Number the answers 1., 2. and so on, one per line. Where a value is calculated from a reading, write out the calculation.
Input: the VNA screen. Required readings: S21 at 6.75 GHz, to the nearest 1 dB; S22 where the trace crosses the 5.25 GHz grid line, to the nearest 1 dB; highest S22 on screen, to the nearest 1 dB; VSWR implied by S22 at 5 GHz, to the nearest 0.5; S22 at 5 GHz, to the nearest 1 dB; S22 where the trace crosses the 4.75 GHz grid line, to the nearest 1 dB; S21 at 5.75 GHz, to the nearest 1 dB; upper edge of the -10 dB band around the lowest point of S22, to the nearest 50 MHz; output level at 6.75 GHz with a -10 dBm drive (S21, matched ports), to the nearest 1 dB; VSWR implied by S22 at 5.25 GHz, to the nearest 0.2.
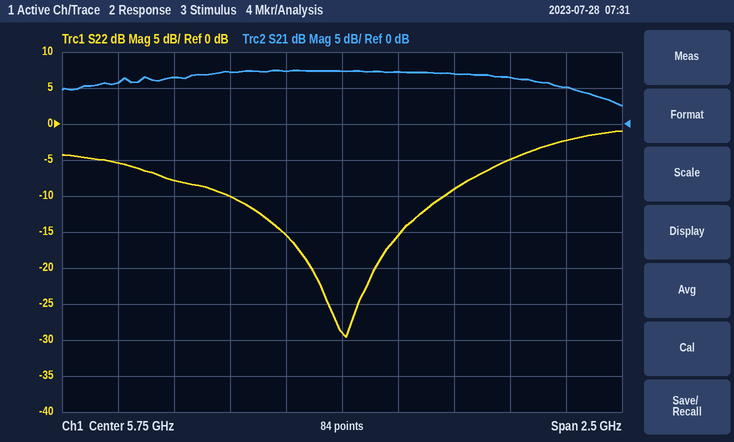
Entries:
1. 5 dB
2. -10 dB
3. -1 dB
4. |Γ| = 10^(-8/20) = 0.3981; VSWR = (1 + 0.3981)/(1 − 0.3981) ≈ 2.32, so 2.5 to the nearest 0.5
5. -8 dB
6. -5 dB
7. 7 dB
8. 6.20 GHz
9. -10 dBm + (5 dB) = -5 dBm
10. |Γ| = 10^(-10/20) = 0.3162; VSWR = (1 + 0.3162)/(1 − 0.3162) ≈ 1.92, so 2.0 to the nearest 0.2
